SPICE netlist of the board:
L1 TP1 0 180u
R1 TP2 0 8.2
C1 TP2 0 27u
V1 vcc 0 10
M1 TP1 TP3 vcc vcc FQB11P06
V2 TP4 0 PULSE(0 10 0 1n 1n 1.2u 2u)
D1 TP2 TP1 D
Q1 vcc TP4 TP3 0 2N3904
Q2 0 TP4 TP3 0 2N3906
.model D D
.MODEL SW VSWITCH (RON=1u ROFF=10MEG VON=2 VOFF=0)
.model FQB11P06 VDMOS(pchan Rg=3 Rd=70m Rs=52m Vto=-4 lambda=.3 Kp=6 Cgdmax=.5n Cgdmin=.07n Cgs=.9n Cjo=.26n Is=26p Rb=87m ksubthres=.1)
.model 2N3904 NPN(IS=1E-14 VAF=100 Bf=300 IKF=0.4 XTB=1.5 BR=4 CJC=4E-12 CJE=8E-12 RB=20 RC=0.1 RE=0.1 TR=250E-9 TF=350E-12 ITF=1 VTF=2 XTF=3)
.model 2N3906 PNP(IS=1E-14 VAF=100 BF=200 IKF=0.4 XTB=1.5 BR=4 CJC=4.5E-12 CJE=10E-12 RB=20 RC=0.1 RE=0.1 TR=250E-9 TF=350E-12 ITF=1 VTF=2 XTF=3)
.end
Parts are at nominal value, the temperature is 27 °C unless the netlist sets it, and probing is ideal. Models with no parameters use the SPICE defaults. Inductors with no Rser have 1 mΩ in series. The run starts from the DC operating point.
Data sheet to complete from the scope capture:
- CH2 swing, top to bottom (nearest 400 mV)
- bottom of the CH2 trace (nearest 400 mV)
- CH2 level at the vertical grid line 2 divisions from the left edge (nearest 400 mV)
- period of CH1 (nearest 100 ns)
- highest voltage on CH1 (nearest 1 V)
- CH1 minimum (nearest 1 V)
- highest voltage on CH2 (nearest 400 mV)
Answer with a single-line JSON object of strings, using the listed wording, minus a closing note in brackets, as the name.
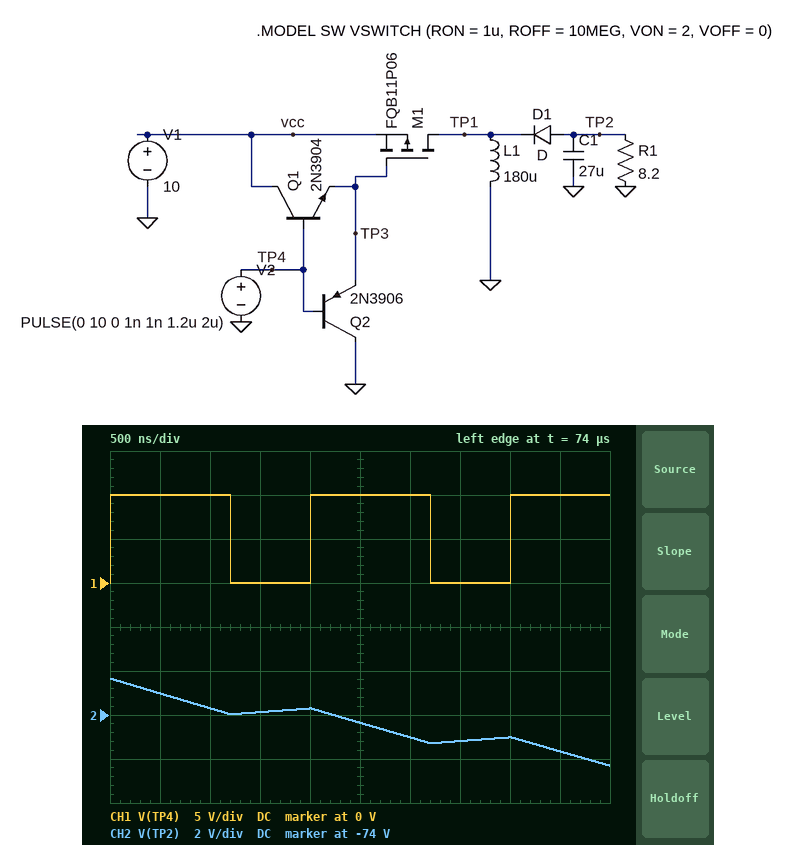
{"CH2 swing, top to bottom": "4.0 V", "bottom of the CH2 trace": "-76.4 V", "CH2 level at the vertical grid line 2 divisions from the left edge": "-73.6 V", "period of CH1": "2.0 µs", "highest voltage on CH1": "10 V", "CH1 minimum": "0 V", "highest voltage on CH2": "-72.4 V"}
